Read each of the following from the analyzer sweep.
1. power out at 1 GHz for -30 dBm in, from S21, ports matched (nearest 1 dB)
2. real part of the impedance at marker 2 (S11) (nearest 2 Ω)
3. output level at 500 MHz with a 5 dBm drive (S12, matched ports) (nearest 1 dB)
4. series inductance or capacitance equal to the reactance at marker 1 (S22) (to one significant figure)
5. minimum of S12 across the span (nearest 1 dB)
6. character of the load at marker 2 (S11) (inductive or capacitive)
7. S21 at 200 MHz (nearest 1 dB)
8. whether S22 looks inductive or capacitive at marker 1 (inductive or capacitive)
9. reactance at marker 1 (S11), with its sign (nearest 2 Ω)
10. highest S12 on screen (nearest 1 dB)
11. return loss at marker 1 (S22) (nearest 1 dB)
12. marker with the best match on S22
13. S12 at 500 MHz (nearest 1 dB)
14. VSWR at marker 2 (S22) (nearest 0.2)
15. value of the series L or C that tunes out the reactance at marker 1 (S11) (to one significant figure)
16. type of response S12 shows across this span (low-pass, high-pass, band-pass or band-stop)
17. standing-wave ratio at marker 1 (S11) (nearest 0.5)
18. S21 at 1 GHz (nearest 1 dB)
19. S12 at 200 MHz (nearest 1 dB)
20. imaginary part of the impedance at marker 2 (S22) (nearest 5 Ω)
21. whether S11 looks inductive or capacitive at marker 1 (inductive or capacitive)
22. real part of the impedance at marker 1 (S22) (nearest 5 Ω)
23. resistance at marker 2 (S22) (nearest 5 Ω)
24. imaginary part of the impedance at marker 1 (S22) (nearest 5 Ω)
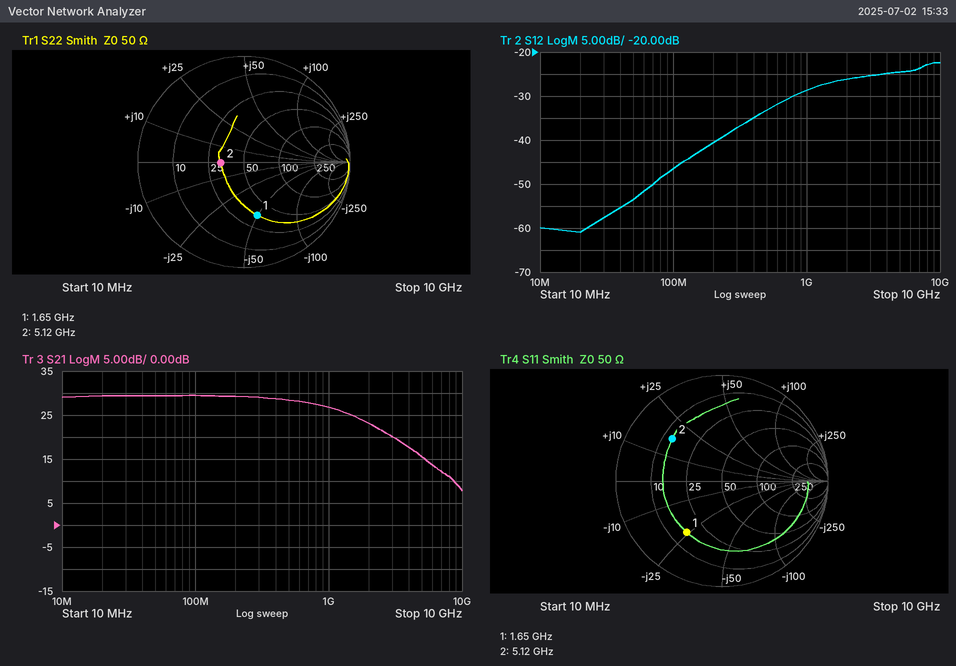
-3 dBm
14 Ω
-28 dBm
2 pF
-61 dB
inductive
29 dB
capacitive
-24 Ω
-22 dB
6 dB
marker 2
-33 dB
1.6
2 nH
high-pass
4.0
27 dB
-41 dB
0 Ω
capacitive
35 Ω
30 Ω
-50 Ω
